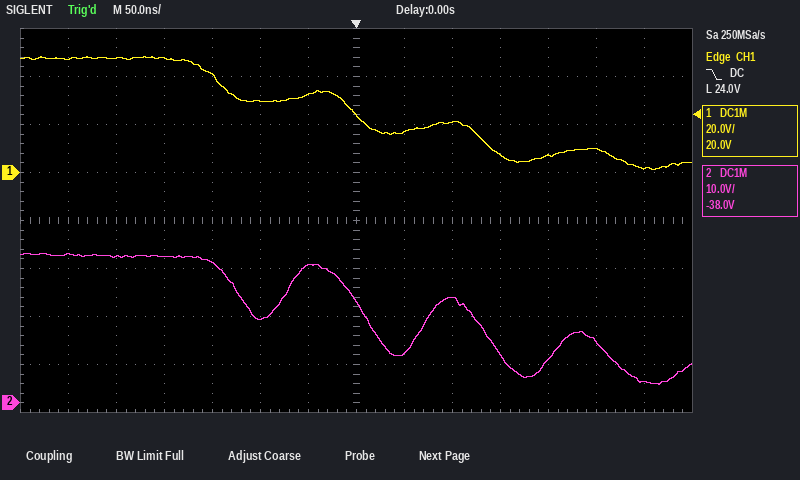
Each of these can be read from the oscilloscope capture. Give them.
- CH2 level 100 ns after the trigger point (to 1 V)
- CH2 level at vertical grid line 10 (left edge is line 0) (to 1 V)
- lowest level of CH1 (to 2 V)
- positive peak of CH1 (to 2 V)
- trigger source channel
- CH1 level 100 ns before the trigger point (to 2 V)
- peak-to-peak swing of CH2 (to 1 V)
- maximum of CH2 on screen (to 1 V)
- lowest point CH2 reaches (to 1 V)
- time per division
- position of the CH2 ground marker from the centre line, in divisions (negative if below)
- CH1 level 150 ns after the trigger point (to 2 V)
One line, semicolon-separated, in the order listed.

22 V; 10 V; 2 V; 48 V; CH1; 30 V; 27 V; 31 V; 4 V; 50 ns; -3.8 div; 8 V
